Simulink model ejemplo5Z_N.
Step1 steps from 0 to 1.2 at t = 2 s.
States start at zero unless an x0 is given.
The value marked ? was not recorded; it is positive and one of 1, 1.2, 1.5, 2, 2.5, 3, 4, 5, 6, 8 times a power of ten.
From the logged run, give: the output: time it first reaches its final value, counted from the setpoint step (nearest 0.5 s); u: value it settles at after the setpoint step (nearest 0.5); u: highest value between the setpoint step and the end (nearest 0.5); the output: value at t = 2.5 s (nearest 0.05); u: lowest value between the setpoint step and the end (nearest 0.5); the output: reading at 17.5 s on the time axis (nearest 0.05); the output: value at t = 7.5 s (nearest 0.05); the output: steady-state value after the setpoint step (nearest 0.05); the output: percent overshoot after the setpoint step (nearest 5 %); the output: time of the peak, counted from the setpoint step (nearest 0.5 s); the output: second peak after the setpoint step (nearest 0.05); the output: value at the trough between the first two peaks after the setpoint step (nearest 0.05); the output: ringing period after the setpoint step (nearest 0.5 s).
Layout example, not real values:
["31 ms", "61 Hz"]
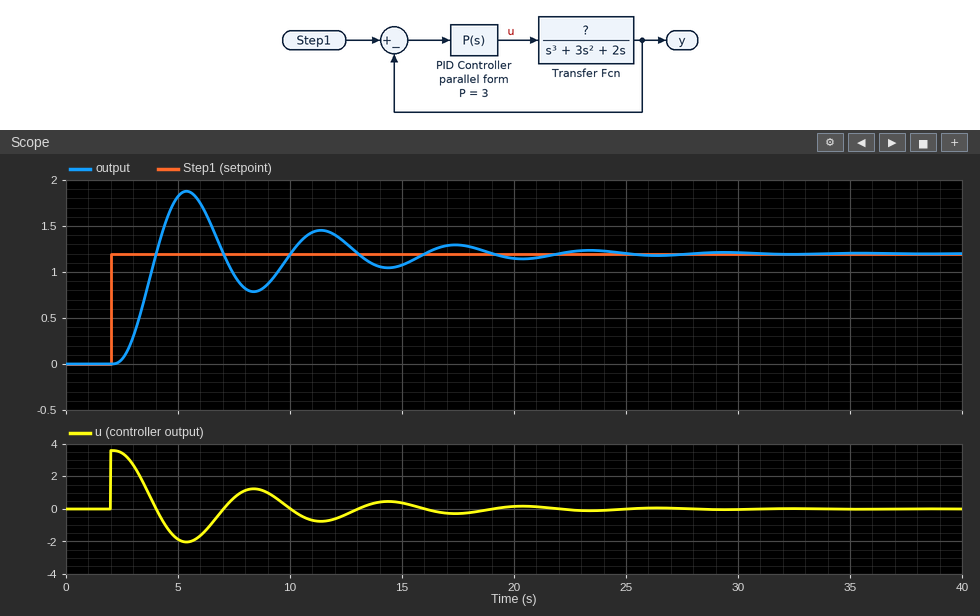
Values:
["2.0 s", "0.0", "3.5", "0.05", "-2.0", "1.30", "0.95", "1.20", "55 %", "3.5 s", "1.45", "0.80", "6.0 s"]
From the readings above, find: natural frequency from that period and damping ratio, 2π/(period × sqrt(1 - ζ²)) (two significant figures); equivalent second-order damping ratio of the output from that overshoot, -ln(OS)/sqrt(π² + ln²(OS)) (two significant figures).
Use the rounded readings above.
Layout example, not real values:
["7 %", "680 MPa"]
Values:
["1.1 rad/s", "0.19"]
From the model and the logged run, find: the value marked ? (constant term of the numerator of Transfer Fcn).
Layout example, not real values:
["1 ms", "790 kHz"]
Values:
["1"]
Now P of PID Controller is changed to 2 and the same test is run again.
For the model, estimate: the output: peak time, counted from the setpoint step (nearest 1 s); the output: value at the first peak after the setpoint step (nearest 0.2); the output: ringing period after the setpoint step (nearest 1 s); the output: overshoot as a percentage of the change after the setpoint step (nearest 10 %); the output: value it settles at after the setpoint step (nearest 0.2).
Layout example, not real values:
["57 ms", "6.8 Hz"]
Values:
["4 s", "1.6", "7 s", "40 %", "1.2"]
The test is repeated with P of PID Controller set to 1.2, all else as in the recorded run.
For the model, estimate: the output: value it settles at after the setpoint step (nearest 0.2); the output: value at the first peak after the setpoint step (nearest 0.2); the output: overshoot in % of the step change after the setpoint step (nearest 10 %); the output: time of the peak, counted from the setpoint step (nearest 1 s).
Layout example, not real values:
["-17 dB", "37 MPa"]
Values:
["1.2", "1.4", "20 %", "5 s"]
